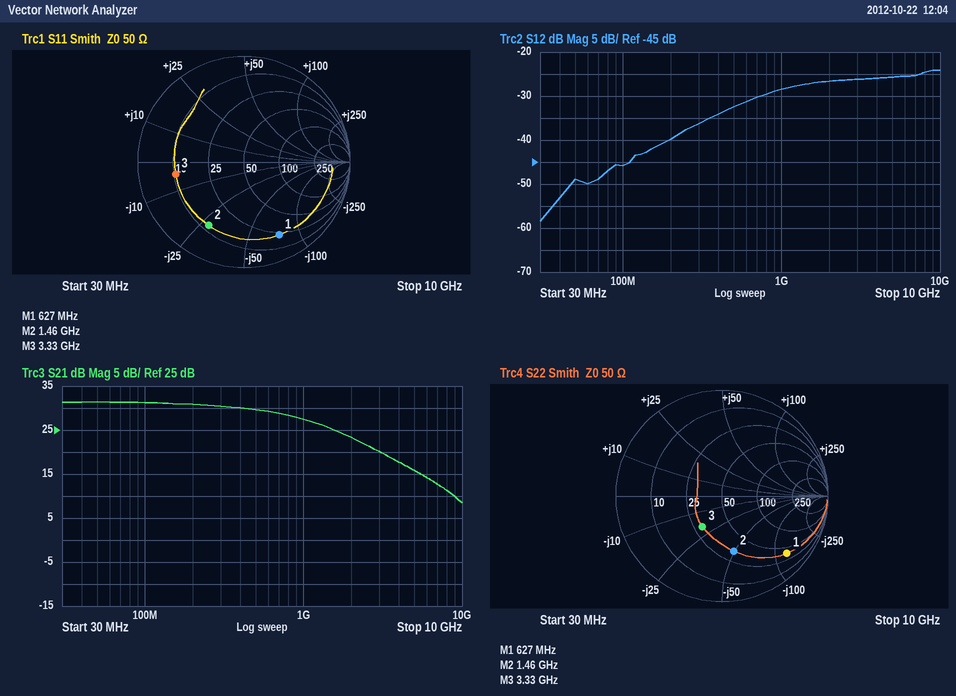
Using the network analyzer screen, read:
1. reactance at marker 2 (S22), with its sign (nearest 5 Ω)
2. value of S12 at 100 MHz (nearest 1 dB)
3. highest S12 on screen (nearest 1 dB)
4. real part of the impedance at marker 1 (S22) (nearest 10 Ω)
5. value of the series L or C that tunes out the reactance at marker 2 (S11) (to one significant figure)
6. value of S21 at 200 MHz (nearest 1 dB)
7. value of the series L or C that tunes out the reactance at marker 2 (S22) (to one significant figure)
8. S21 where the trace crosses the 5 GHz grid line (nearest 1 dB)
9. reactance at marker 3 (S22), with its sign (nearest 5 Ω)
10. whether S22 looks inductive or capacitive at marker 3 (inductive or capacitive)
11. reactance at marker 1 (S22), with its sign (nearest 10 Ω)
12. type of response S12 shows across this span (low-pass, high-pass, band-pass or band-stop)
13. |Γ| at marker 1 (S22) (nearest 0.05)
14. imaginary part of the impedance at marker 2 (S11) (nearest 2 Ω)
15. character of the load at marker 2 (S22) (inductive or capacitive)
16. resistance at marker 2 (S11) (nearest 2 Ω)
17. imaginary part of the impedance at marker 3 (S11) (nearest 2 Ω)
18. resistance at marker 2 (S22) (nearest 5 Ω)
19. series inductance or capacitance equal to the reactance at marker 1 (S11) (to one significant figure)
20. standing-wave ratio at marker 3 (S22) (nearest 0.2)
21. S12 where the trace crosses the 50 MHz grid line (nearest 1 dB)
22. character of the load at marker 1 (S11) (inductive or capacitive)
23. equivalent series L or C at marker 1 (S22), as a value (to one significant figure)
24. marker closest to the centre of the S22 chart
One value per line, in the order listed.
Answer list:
-50 Ω
-46 dB
-24 dB
40 Ω
3 nH
31 dB
5 nH
16 dB
-20 Ω
capacitive
-120 Ω
high-pass
0.80
-28 Ω
capacitive
12 Ω
-4 Ω
35 Ω
3 pF
2.0
-49 dB
capacitive
2 pF
marker 3
